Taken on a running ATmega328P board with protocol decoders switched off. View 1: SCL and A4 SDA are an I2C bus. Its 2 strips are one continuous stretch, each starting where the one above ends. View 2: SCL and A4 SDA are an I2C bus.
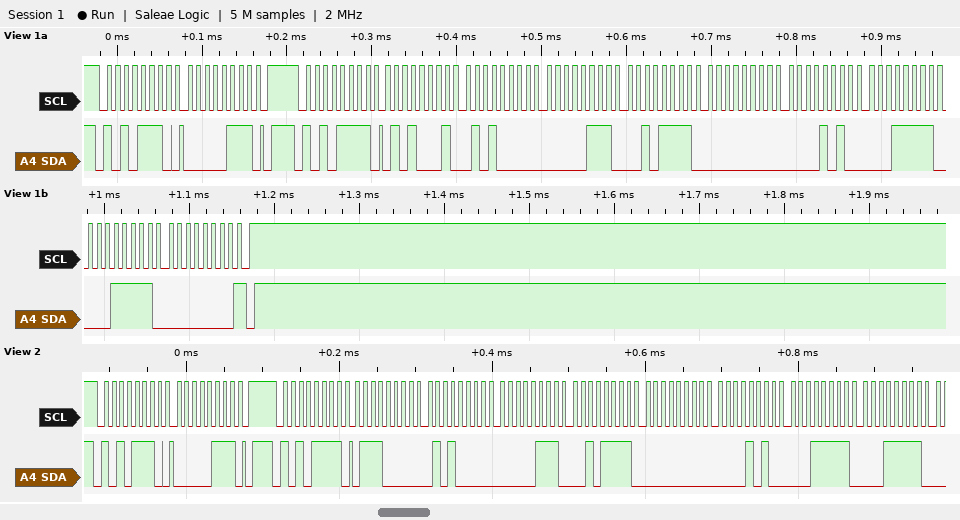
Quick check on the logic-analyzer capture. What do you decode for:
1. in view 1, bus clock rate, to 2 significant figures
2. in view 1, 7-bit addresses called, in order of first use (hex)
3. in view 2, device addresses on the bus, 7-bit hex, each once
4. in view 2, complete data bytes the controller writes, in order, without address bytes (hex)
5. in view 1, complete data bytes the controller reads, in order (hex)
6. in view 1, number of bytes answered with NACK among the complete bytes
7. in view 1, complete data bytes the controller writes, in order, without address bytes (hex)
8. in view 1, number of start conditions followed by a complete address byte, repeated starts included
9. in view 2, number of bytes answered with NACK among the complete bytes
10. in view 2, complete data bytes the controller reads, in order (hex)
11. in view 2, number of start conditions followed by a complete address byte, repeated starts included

100 kHz
0x57
0x57
07
51 50 07 2F 00 0A 1F 1F 00
1
07
2
0
70 50 07 2F 00 0A 1F 1F
2
